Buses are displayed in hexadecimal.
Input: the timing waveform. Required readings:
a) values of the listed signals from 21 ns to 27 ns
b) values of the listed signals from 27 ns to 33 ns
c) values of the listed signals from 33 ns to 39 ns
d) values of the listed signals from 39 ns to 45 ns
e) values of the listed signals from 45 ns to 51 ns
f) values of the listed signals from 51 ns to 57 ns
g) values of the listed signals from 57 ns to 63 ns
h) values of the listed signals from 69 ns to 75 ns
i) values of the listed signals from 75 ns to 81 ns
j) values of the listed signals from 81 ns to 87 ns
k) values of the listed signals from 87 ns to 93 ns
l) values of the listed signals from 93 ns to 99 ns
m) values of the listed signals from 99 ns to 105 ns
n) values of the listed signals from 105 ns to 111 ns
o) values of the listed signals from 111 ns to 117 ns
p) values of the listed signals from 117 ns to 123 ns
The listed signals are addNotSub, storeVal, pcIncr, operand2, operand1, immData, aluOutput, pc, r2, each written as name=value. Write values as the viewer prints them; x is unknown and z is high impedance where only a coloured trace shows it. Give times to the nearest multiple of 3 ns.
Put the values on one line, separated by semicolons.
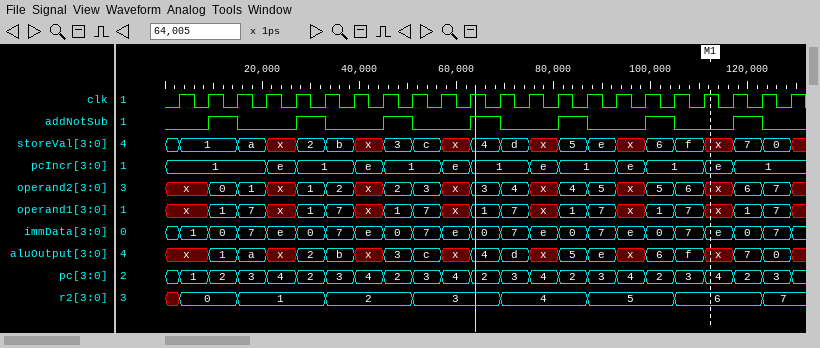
addNotSub=0, storeVal=x, pcIncr=e, operand2=x, operand1=x, immData=e, aluOutput=x, pc=4, r2=1; addNotSub=1, storeVal=2, pcIncr=1, operand2=1, operand1=1, immData=0, aluOutput=2, pc=2, r2=1; addNotSub=0, storeVal=b, pcIncr=1, operand2=2, operand1=7, immData=7, aluOutput=b, pc=3, r2=2; addNotSub=0, storeVal=x, pcIncr=e, operand2=x, operand1=x, immData=e, aluOutput=x, pc=4, r2=2; addNotSub=1, storeVal=3, pcIncr=1, operand2=2, operand1=1, immData=0, aluOutput=3, pc=2, r2=2; addNotSub=0, storeVal=c, pcIncr=1, operand2=3, operand1=7, immData=7, aluOutput=c, pc=3, r2=3; addNotSub=0, storeVal=x, pcIncr=e, operand2=x, operand1=x, immData=e, aluOutput=x, pc=4, r2=3; addNotSub=0, storeVal=d, pcIncr=1, operand2=4, operand1=7, immData=7, aluOutput=d, pc=3, r2=4; addNotSub=0, storeVal=x, pcIncr=e, operand2=x, operand1=x, immData=e, aluOutput=x, pc=4, r2=4; addNotSub=1, storeVal=5, pcIncr=1, operand2=4, operand1=1, immData=0, aluOutput=5, pc=2, r2=4; addNotSub=0, storeVal=e, pcIncr=1, operand2=5, operand1=7, immData=7, aluOutput=e, pc=3, r2=5; addNotSub=0, storeVal=x, pcIncr=e, operand2=x, operand1=x, immData=e, aluOutput=x, pc=4, r2=5; addNotSub=1, storeVal=6, pcIncr=1, operand2=5, operand1=1, immData=0, aluOutput=6, pc=2, r2=5; addNotSub=0, storeVal=f, pcIncr=1, operand2=6, operand1=7, immData=7, aluOutput=f, pc=3, r2=6; addNotSub=0, storeVal=x, pcIncr=e, operand2=x, operand1=x, immData=e, aluOutput=x, pc=4, r2=6; addNotSub=1, storeVal=7, pcIncr=1, operand2=6, operand1=1, immData=0, aluOutput=7, pc=2, r2=6
